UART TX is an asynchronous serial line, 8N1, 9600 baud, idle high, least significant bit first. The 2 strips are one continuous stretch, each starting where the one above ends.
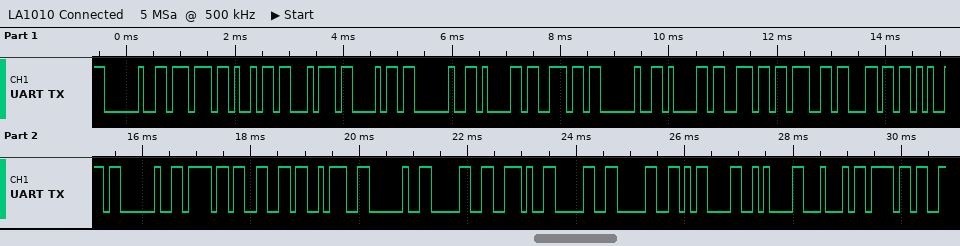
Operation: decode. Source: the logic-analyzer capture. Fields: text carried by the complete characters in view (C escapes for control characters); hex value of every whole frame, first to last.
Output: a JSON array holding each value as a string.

["\" with an angle of: 0.00\\r\\nDo\"", "20 77 69 74 68 20 61 6E 20 61 6E 67 6C 65 20 6F 66 3A 20 30 2E 30 30 0D 0A 44 6F"]
